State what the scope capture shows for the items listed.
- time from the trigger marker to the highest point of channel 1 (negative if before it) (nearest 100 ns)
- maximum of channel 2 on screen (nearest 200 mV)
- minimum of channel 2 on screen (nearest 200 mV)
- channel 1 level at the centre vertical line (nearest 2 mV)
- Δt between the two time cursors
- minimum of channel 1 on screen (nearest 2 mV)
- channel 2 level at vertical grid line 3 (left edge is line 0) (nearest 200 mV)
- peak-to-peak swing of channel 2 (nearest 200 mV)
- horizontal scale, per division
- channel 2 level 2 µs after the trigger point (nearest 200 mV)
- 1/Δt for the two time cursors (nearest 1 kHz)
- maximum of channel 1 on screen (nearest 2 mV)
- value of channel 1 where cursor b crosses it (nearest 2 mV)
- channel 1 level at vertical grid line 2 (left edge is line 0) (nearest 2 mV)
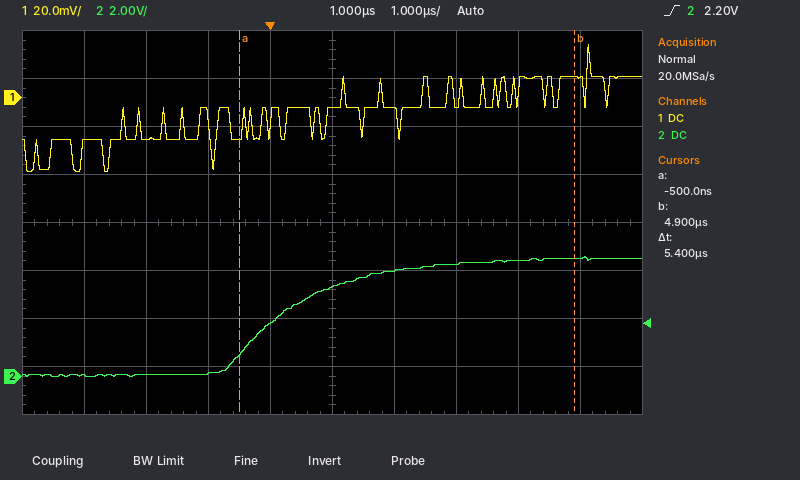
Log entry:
+5.1 µs
5.0 V
0.0 V
-4 mV
5.4 µs
-30 mV
200 mV
5.0 V
1 µs
4.4 V
185 kHz
22 mV
8 mV
-18 mV
